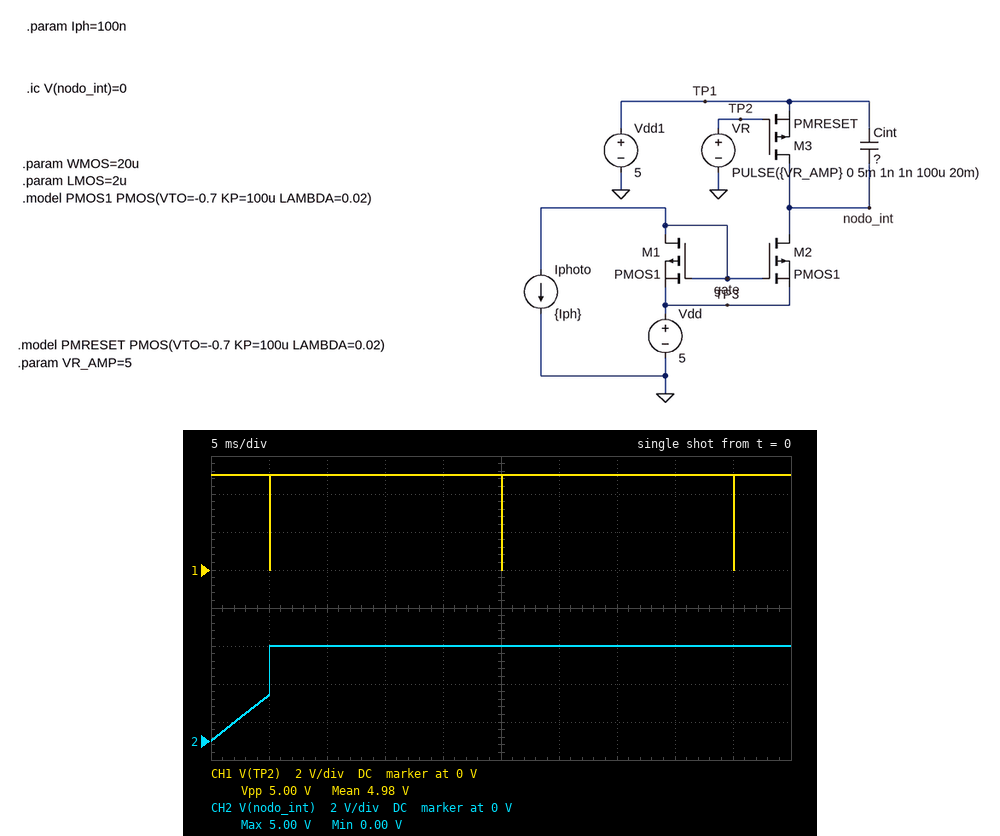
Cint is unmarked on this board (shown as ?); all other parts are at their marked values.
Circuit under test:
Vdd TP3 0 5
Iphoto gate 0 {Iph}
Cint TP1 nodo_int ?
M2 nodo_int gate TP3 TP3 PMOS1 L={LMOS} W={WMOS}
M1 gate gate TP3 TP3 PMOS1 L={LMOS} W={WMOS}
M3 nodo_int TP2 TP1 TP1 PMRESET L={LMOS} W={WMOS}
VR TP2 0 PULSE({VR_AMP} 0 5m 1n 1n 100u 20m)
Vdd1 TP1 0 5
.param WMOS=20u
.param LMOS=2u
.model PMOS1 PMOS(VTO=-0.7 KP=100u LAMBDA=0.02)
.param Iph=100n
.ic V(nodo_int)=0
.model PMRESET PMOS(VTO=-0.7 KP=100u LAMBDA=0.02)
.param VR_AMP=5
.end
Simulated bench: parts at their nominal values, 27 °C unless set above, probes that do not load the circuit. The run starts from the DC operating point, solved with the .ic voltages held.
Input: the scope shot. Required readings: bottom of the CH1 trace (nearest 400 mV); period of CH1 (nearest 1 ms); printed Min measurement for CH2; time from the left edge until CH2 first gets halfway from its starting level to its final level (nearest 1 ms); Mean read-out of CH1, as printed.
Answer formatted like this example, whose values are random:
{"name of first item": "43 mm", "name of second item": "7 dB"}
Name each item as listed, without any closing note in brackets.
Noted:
{"bottom of the CH1 trace": "0 V", "period of CH1": "20 ms", "printed Min measurement for CH2": "0.00 V", "time from the left edge until CH2 first gets halfway from its starting level to its final level": "5 ms", "Mean read-out of CH1, as printed": "4.98 V"}
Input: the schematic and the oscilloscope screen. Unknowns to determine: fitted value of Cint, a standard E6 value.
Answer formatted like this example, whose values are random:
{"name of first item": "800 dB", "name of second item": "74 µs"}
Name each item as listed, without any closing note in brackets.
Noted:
{"fitted value of Cint, a standard E6 value": "220 pF"}
